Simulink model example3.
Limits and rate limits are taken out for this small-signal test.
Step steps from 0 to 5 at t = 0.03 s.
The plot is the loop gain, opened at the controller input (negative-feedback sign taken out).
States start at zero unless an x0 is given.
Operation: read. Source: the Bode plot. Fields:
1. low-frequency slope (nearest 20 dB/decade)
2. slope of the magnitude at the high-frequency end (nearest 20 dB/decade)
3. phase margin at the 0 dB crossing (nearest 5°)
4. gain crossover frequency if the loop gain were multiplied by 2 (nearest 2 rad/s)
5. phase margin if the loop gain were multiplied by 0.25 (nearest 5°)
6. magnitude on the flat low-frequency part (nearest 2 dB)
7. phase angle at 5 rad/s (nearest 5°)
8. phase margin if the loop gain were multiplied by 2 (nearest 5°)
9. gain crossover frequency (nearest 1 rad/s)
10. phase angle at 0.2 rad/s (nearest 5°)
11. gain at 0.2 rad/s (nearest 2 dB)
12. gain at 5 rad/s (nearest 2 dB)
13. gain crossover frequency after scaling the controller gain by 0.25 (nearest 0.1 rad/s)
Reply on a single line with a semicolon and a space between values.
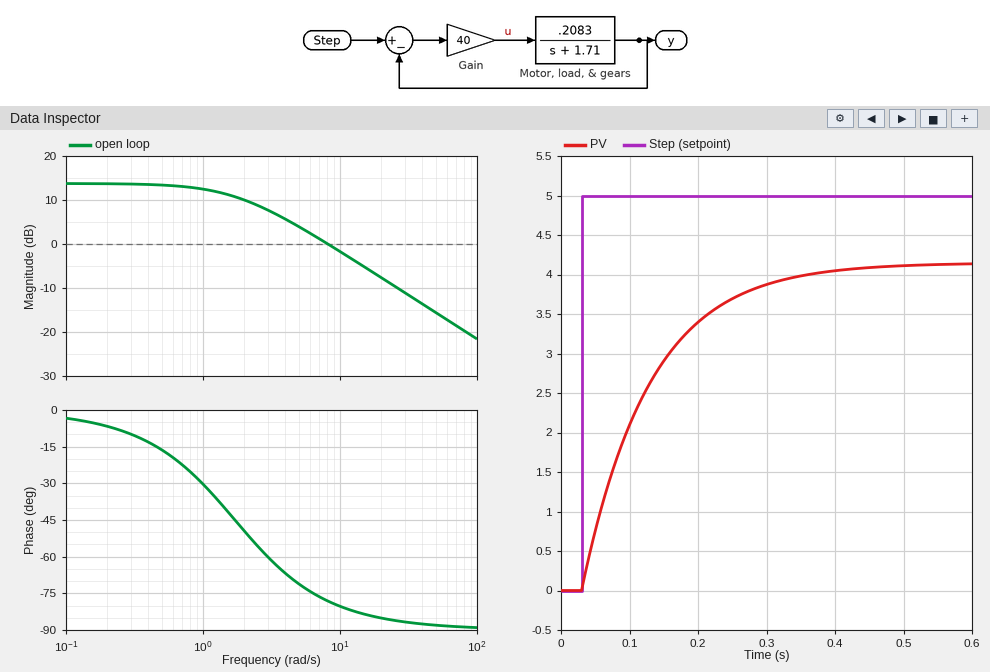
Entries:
0 dB/decade; -20 dB/decade; 100°; 16 rad/s; 145°; 14 dB; -70°; 95°; 8 rad/s; -5°; 14 dB; 4 dB; 1.2 rad/s
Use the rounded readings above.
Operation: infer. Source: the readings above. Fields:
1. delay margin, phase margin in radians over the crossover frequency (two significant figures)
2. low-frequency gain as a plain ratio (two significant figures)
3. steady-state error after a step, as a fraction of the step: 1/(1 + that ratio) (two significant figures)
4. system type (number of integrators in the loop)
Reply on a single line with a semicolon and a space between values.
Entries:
0.22 s; 5.0; 0.17; 0
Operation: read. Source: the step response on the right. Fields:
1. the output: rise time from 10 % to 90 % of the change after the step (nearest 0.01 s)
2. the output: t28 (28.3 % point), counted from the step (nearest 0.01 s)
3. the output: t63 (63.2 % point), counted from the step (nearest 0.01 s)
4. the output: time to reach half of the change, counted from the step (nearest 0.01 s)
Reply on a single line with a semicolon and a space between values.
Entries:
0.22 s; 0.03 s; 0.10 s; 0.07 s
